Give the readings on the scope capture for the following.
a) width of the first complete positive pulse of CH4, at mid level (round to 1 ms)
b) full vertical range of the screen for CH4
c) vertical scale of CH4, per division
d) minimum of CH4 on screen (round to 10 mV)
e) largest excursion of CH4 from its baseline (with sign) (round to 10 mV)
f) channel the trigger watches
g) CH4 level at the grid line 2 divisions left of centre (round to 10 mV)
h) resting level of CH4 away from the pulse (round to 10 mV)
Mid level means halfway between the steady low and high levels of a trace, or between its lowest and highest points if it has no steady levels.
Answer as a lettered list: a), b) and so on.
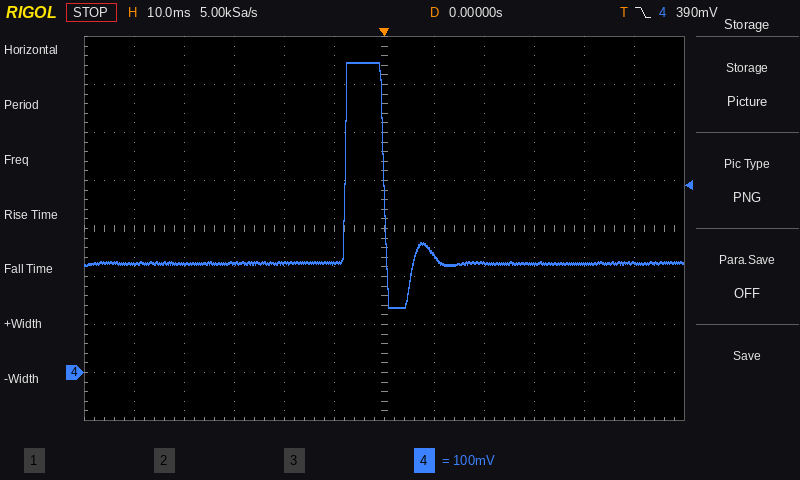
a) 8 ms
b) 800 mV
c) 100 mV
d) 140 mV
e) +420 mV
f) CH4
g) 230 mV
h) 230 mV
